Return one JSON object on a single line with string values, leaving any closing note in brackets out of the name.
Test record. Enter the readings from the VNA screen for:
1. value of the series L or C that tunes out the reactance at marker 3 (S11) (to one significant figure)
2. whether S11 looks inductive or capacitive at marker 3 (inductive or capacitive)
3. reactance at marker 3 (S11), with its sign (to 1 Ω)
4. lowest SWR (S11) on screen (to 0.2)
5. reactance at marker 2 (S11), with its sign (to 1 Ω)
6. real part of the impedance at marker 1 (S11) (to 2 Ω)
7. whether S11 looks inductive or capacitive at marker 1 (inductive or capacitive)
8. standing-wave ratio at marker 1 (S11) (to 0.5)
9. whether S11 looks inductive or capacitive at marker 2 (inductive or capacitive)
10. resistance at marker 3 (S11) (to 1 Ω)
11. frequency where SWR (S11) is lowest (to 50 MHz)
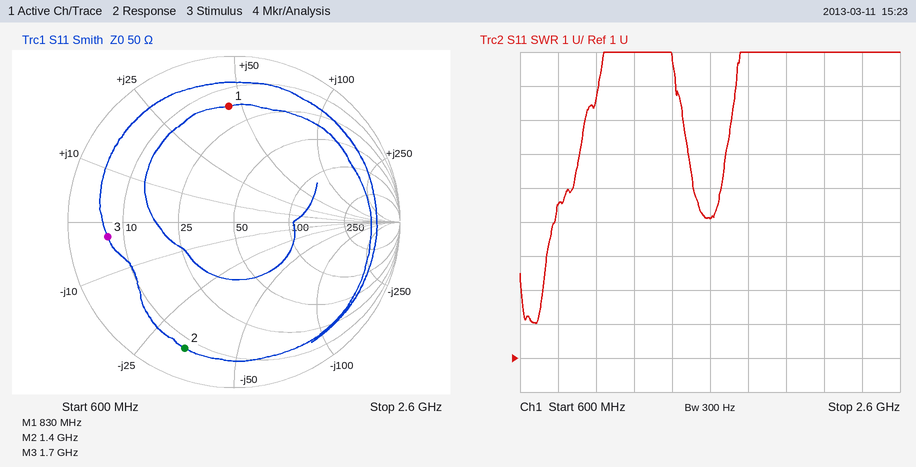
{"value of the series L or C that tunes out the reactance at marker 3 (S11)": "300 pH", "whether S11 looks inductive or capacitive at marker 3": "capacitive", "reactance at marker 3 (S11), with its sign": "-3 Ω", "lowest SWR (S11) on screen": "2.0", "reactance at marker 2 (S11), with its sign": "-34 Ω", "real part of the impedance at marker 1 (S11)": "16 Ω", "whether S11 looks inductive or capacitive at marker 1": "inductive", "standing-wave ratio at marker 1 (S11)": "5.5", "whether S11 looks inductive or capacitive at marker 2": "capacitive", "resistance at marker 3 (S11)": "7 Ω", "frequency where SWR (S11) is lowest": "700 MHz"}
